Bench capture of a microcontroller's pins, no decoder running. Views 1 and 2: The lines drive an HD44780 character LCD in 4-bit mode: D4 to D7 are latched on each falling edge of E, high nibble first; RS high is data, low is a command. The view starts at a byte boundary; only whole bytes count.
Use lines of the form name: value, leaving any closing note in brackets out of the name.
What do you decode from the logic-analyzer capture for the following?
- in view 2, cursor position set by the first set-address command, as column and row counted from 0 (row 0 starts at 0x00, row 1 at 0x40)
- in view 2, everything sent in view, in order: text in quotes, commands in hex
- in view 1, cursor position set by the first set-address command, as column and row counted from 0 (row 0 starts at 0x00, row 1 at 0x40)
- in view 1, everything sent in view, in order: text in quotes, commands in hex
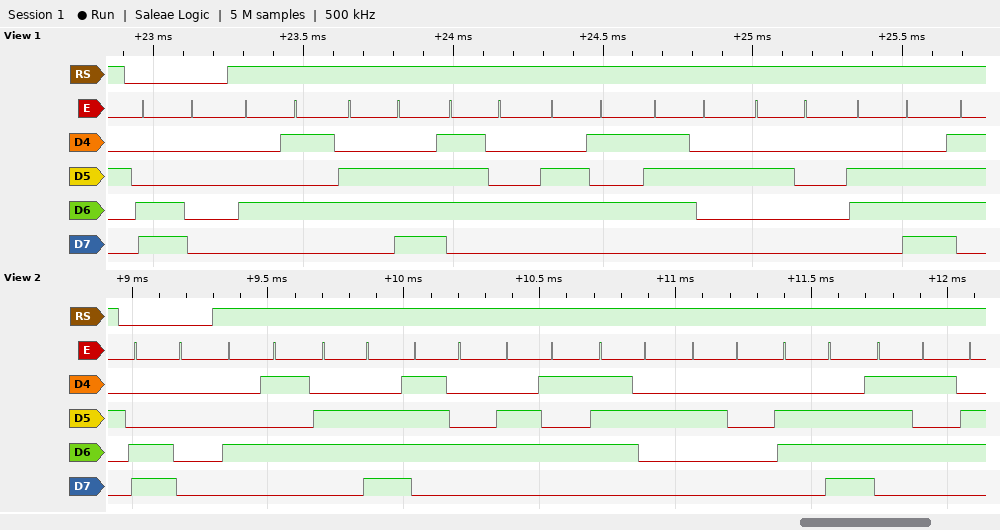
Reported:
in view 2, cursor position set by the first set-address command, as column and row counted from 0: column 0, row 1
in view 2, everything sent in view, in order: text in quotes, commands in hex: 0xC0 "Enter nu"
in view 1, cursor position set by the first set-address command, as column and row counted from 0: column 0, row 1
in view 1, everything sent in view, in order: text in quotes, commands in hex: 0xC0 "Enter n"
